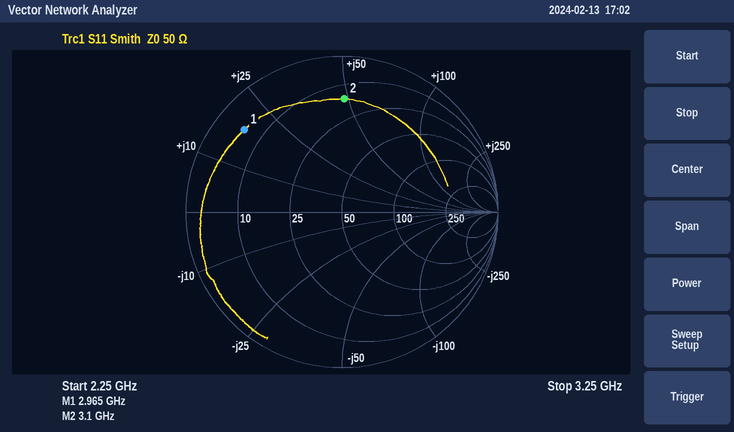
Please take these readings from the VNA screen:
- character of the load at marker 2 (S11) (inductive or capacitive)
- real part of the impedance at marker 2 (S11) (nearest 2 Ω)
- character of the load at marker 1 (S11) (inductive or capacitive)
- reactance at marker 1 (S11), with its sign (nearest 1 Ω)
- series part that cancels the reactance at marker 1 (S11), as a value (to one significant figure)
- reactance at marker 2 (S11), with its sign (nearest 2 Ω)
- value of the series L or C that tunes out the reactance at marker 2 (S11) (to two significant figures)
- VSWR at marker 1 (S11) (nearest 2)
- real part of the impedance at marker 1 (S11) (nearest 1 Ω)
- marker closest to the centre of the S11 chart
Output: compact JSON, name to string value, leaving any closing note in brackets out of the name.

{"character of the load at marker 2 (S11)": "inductive", "real part of the impedance at marker 2 (S11)": "16 Ω", "character of the load at marker 1 (S11)": "inductive", "reactance at marker 1 (S11), with its sign": "+18 Ω", "series part that cancels the reactance at marker 1 (S11), as a value": "3 pF", "reactance at marker 2 (S11), with its sign": "+48 Ω", "value of the series L or C that tunes out the reactance at marker 2 (S11)": "1.1 pF", "VSWR at marker 1 (S11)": "10", "real part of the impedance at marker 1 (S11)": "6 Ω", "marker closest to the centre of the S11 chart": "marker 2"}
